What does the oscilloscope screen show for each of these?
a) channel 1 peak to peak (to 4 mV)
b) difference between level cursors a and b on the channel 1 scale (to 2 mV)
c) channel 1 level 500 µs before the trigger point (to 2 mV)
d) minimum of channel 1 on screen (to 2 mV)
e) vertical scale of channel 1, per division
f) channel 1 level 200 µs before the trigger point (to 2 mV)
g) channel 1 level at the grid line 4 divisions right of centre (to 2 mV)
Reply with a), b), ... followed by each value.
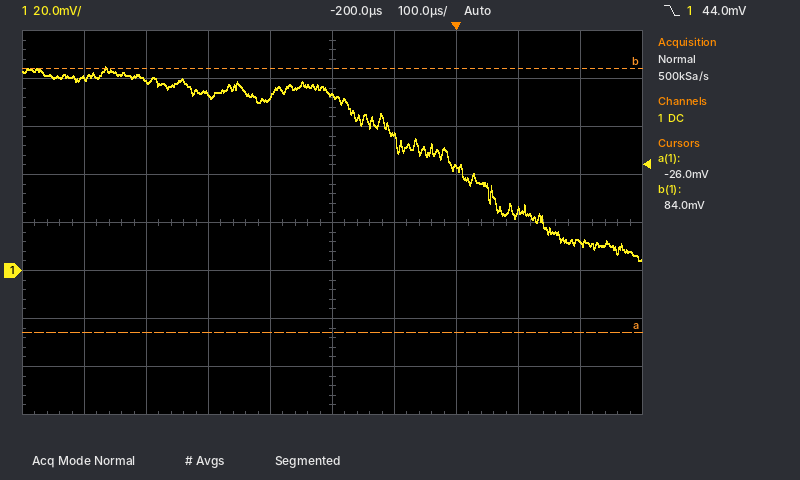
a) 80 mV
b) 110 mV
c) 80 mV
d) 4 mV
e) 20 mV
f) 72 mV
g) 12 mV
